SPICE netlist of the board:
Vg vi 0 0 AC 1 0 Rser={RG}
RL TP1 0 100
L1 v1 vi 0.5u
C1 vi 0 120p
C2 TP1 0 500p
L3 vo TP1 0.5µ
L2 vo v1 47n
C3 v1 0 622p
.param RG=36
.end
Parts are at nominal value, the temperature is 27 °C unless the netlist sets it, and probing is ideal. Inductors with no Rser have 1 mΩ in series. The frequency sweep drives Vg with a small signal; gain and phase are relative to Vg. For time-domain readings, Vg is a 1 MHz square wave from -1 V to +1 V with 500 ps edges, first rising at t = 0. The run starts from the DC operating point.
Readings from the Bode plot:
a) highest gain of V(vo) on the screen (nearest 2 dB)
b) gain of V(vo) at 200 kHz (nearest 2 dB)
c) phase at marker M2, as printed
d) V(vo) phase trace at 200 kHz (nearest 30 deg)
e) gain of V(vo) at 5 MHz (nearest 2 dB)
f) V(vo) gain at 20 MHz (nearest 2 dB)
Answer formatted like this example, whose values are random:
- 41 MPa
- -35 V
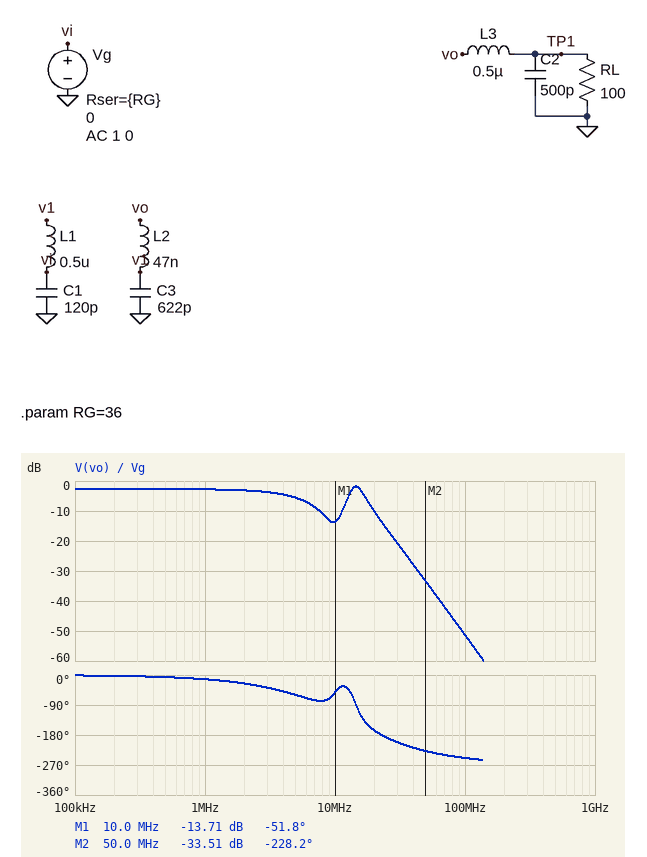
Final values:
- -2 dB
- -2 dB
- -228.2 deg
- 0 deg
- -6 dB
- -10 dB
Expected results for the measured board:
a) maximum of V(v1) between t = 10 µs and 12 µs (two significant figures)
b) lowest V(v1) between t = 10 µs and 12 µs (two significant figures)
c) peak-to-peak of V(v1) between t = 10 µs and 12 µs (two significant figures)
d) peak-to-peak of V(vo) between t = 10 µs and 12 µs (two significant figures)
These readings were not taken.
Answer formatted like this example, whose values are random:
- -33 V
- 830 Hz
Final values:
- 890 mV
- -890 mV
- 1.8 V
- 1.7 V
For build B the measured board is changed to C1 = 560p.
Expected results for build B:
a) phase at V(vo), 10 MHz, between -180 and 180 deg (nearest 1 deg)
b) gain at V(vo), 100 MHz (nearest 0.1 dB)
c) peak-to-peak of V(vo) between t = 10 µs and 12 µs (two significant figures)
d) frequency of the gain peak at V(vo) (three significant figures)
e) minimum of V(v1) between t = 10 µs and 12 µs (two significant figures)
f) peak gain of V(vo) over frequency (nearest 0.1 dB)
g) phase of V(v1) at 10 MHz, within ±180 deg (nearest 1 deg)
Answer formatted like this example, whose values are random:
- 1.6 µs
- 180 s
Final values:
- -91 deg
- -64.4 dB
- 1.6 V
- 15.4 MHz
- -830 mV
- 1.0 dB
- -76 deg
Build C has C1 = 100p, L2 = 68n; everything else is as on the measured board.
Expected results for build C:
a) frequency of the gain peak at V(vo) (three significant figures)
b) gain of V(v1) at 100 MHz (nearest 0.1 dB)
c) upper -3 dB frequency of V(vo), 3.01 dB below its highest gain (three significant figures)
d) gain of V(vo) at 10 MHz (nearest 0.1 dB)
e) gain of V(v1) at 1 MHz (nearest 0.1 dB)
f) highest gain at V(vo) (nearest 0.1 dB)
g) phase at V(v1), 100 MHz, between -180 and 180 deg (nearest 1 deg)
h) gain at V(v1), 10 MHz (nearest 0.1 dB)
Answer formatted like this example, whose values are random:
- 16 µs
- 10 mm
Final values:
- 14.2 MHz
- -49.1 dB
- 16.5 MHz
- -13.6 dB
- -2.8 dB
- -2.4 dB
- 115 deg
- -12.1 dB
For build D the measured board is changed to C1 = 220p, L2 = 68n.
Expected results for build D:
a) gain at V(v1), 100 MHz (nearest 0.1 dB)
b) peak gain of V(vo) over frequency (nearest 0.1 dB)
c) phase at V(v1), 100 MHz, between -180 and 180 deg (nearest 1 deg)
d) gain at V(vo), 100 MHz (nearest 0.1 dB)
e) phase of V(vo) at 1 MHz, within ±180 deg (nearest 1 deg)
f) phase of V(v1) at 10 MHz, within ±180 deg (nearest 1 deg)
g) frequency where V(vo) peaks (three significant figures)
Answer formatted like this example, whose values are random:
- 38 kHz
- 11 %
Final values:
- -55.6 dB
- -2.0 dB
- 102 deg
- -56.7 dB
- -14 deg
- -41 deg
- 14.9 MHz
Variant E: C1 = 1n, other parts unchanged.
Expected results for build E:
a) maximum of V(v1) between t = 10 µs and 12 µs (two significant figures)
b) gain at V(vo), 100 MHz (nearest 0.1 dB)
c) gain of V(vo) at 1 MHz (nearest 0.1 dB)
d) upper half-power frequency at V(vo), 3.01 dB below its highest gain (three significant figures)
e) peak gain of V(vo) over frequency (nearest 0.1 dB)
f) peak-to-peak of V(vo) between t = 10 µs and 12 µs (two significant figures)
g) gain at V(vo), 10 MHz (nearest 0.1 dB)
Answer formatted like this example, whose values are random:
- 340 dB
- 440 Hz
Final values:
- 810 mV
- -69.5 dB
- -3.1 dB
- 15.6 MHz
- 0.1 dB
- 1.6 V
- -15.5 dB
